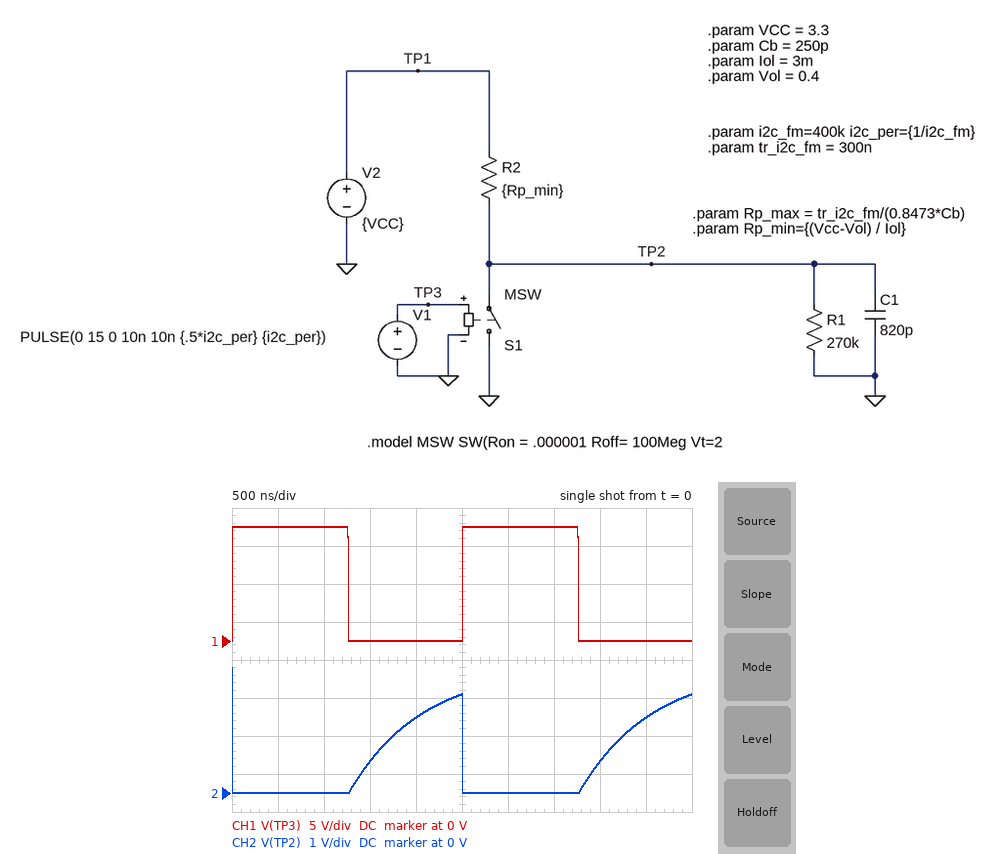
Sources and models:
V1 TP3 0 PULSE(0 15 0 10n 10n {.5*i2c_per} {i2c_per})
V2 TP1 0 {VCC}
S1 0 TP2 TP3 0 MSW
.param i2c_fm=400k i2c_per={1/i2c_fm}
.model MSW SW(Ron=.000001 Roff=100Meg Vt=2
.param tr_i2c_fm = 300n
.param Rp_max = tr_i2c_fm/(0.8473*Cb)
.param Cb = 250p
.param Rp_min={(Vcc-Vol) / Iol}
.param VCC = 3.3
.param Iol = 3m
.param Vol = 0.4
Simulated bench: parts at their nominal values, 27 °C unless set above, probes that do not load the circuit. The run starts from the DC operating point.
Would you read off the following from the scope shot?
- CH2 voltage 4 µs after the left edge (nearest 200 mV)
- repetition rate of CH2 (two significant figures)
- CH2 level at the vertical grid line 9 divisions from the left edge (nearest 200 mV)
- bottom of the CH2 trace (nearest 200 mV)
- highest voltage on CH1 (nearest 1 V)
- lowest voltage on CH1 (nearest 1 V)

800 mV
400 kHz
2.0 V
0 V
15 V
0 V
